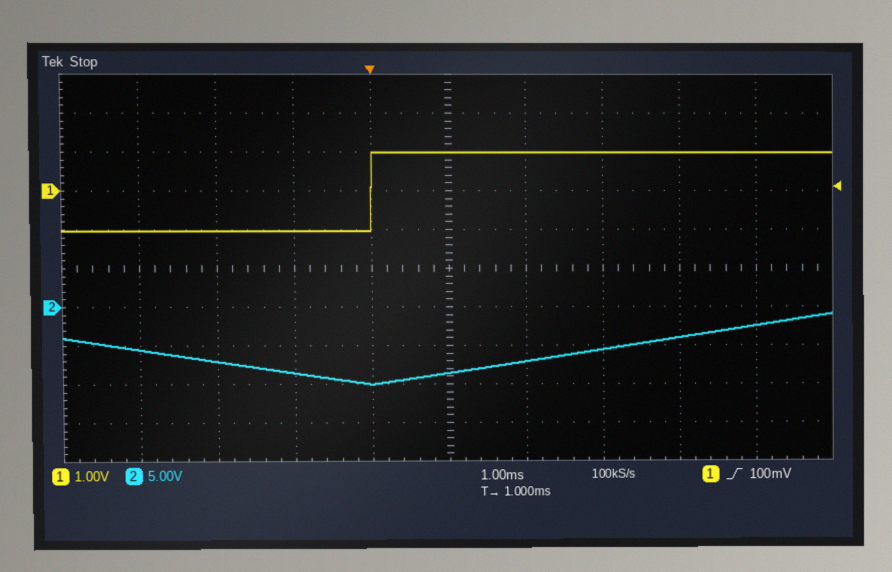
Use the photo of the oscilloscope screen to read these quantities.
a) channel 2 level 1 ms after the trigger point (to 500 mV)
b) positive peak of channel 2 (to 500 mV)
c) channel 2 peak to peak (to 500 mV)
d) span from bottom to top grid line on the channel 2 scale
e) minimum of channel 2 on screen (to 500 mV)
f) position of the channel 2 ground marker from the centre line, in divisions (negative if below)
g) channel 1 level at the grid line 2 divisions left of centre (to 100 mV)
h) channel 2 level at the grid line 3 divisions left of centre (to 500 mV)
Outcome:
-8.5 V
-1.0 V
9.0 V
50 V
-10.0 V
-1.0 div
-1.0 V
-7.0 V
